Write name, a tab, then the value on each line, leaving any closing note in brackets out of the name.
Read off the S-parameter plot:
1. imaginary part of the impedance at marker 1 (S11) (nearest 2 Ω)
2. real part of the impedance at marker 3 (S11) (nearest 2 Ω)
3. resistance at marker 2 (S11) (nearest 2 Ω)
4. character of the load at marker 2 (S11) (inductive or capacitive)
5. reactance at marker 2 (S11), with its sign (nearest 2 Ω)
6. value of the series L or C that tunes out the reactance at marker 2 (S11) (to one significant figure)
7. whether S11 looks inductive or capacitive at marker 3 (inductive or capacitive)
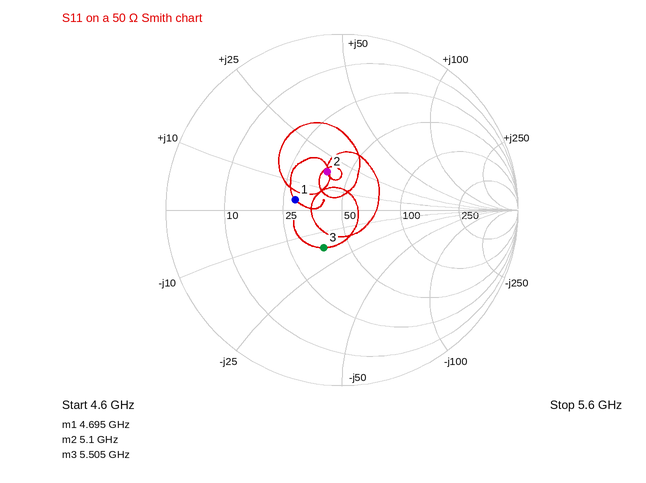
imaginary part of the impedance at marker 1 (S11)	+4 Ω
real part of the impedance at marker 3 (S11)	38 Ω
resistance at marker 2 (S11)	38 Ω
character of the load at marker 2 (S11)	inductive
reactance at marker 2 (S11), with its sign	+18 Ω
value of the series L or C that tunes out the reactance at marker 2 (S11)	2 pF
whether S11 looks inductive or capacitive at marker 3	capacitive
